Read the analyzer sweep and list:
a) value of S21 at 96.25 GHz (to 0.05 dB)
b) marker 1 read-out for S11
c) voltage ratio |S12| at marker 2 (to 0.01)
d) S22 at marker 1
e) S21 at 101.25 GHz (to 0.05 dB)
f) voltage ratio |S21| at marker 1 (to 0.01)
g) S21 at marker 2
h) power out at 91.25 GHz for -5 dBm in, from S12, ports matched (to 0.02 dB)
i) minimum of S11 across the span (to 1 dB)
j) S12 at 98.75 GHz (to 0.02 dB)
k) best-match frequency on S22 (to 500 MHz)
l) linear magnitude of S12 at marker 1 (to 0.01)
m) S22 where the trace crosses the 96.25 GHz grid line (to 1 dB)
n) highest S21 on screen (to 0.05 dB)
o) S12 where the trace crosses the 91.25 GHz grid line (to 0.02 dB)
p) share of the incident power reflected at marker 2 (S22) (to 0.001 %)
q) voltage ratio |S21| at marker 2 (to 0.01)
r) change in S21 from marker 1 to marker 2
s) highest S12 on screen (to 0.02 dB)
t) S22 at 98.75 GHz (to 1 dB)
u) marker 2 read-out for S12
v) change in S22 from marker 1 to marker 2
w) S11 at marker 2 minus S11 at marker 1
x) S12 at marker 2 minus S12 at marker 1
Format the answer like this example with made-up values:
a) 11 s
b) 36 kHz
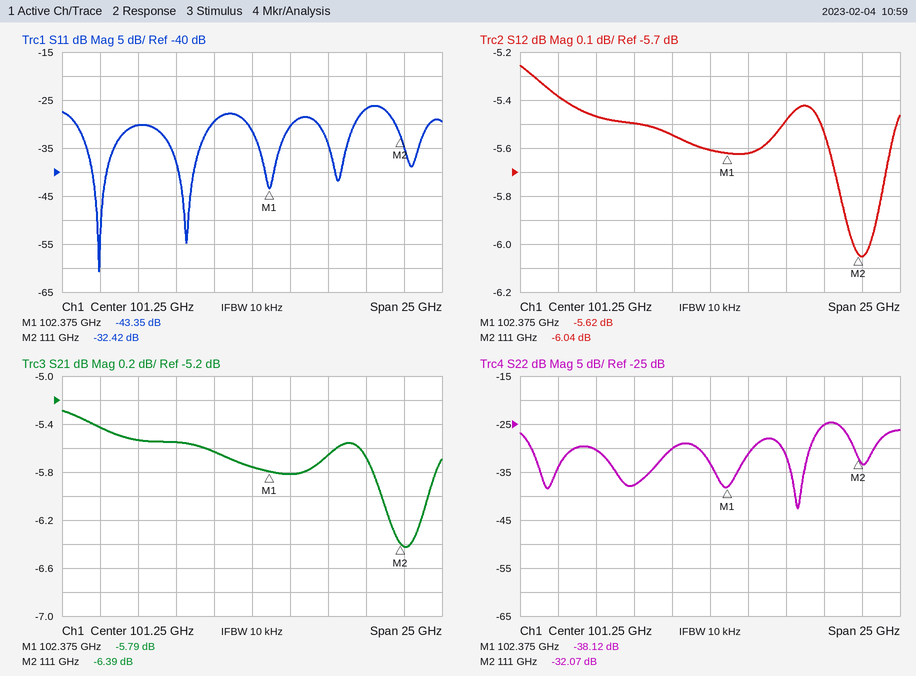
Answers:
a) -5.55 dB
b) -43.35 dB
c) 0.50
d) -38.12 dB
e) -5.75 dB
f) 0.51
g) -6.39 dB
h) -10.38 dBm
i) -61 dB
j) -5.54 dB
k) 107.0 GHz
l) 0.52
m) -38 dB
n) -5.30 dB
o) -5.38 dB
p) 0.062 %
q) 0.48
r) -0.60 dB
s) -5.26 dB
t) -30 dB
u) -6.04 dB
v) 6.05 dB
w) 10.93 dB
x) -0.42 dB
